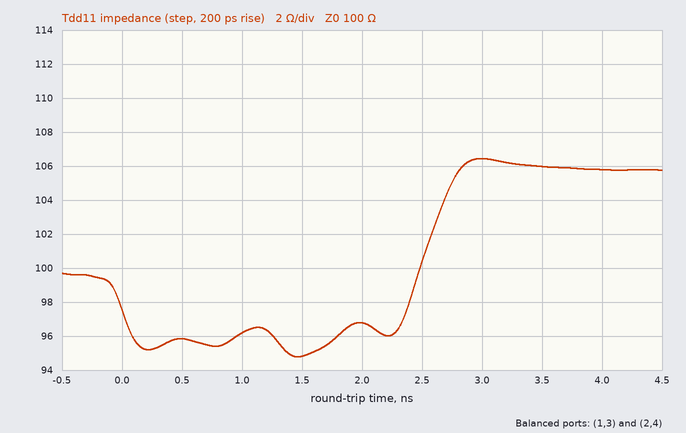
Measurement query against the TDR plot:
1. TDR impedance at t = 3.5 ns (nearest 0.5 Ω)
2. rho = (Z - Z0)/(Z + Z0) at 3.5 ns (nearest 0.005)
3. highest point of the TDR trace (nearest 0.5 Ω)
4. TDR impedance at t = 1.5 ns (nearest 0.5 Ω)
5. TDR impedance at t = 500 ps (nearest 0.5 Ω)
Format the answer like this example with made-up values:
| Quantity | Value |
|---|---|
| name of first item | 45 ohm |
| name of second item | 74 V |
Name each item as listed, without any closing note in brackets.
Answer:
| Quantity | Value |
|---|---|
| TDR impedance at t = 3.5 ns | 106.0 Ω |
| rho = (Z - Z0)/(Z + Z0) at 3.5 ns | +0.030 |
| highest point of the TDR trace | 106.5 Ω |
| TDR impedance at t = 1.5 ns | 95.0 Ω |
| TDR impedance at t = 500 ps | 96.0 Ω |
